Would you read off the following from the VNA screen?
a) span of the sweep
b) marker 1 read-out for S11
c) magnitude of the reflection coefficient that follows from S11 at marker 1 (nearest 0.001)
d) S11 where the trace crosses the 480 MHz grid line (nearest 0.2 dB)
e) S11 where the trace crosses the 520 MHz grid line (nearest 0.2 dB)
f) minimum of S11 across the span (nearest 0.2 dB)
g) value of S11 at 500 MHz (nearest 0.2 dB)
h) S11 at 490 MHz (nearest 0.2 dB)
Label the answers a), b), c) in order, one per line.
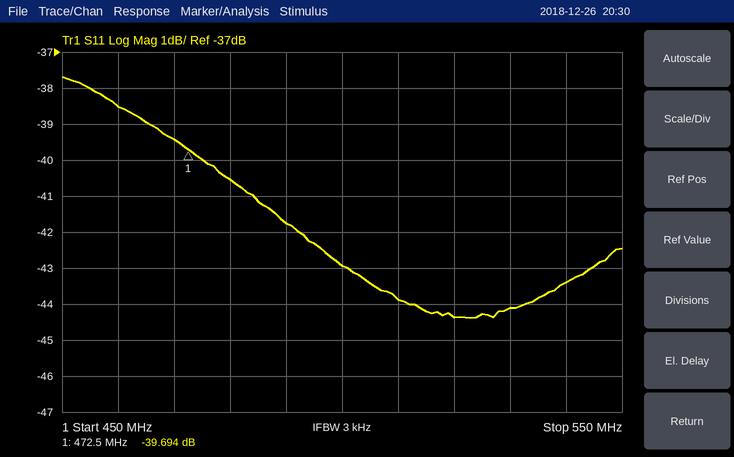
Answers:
a) 100 MHz
b) -39.694 dB
c) 0.010
d) -40.6 dB
e) -44.4 dB
f) -44.4 dB
g) -43.0 dB
h) -41.8 dB
